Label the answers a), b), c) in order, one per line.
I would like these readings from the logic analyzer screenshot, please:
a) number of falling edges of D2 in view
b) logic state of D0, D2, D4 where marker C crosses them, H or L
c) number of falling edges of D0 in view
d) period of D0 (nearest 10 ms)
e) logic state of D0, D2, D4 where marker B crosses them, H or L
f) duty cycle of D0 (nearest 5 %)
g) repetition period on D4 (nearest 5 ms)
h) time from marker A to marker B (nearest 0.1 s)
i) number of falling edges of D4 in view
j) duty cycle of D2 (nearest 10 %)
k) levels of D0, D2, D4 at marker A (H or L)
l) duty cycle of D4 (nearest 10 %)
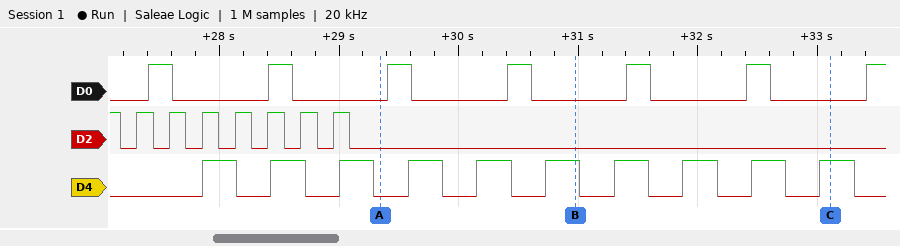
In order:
a) 8
b) D0=L, D2=L, D4=H
c) 6
d) 1000 ms
e) D0=L, D2=L, D4=H
f) 20 %
g) 575 ms
h) 1.6 s
i) 10
j) 50 %
k) D0=L, D2=L, D4=L
l) 50 %
